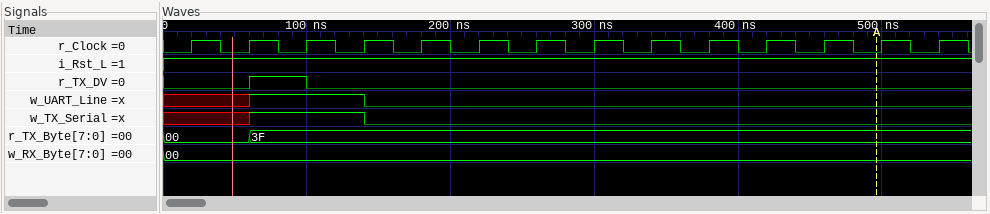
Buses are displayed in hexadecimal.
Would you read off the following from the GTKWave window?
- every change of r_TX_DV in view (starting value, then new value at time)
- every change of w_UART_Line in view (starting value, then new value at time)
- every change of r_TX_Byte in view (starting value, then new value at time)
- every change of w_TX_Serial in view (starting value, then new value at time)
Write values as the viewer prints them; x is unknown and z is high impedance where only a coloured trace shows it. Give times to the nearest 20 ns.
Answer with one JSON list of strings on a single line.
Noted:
["0, 1 at 60 ns, 0 at 100 ns", "x, 1 at 60 ns, 0 at 140 ns", "00, 3F at 60 ns", "x, 1 at 60 ns, 0 at 140 ns"]
